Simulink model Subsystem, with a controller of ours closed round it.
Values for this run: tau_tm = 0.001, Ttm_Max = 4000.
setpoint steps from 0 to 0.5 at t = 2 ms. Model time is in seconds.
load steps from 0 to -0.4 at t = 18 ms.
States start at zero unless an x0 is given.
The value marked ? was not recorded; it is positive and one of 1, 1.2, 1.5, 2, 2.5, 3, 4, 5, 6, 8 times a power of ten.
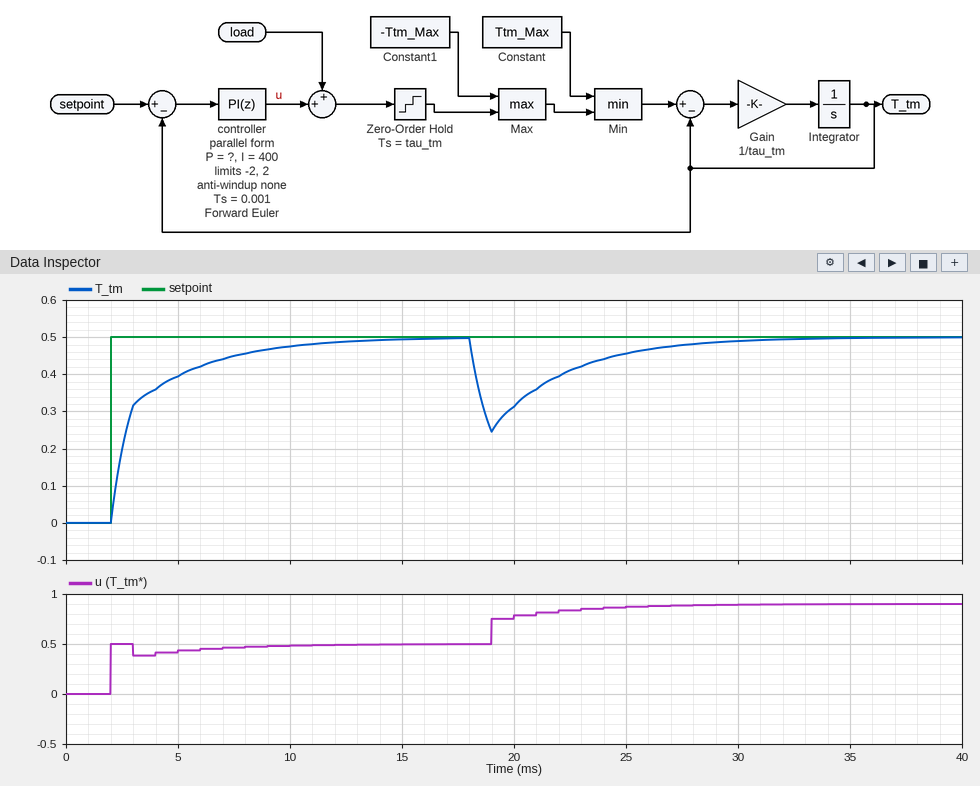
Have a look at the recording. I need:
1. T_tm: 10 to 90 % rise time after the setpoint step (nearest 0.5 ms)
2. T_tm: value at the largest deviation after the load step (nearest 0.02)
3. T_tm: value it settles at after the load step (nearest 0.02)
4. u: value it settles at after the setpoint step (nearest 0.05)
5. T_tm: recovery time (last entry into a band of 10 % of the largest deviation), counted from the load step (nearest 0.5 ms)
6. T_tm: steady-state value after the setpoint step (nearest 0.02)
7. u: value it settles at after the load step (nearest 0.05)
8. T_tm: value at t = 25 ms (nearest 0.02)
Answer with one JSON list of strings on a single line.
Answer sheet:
["5.5 ms", "0.24", "0.50", "0.50", "9.0 ms", "0.50", "0.90", "0.46"]
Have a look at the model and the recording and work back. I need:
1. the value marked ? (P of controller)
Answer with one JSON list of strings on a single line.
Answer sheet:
["1"]
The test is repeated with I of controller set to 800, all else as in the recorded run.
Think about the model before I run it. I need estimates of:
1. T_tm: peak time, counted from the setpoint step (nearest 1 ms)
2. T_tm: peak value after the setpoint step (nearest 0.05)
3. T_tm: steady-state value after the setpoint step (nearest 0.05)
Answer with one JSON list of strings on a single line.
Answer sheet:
["3 ms", "0.55", "0.50"]
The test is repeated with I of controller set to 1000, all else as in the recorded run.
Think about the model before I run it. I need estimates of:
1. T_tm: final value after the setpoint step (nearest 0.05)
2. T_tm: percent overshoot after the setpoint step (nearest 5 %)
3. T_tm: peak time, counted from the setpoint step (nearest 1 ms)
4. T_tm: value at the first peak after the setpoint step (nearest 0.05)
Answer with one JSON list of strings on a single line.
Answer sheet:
["0.50", "20 %", "3 ms", "0.60"]
